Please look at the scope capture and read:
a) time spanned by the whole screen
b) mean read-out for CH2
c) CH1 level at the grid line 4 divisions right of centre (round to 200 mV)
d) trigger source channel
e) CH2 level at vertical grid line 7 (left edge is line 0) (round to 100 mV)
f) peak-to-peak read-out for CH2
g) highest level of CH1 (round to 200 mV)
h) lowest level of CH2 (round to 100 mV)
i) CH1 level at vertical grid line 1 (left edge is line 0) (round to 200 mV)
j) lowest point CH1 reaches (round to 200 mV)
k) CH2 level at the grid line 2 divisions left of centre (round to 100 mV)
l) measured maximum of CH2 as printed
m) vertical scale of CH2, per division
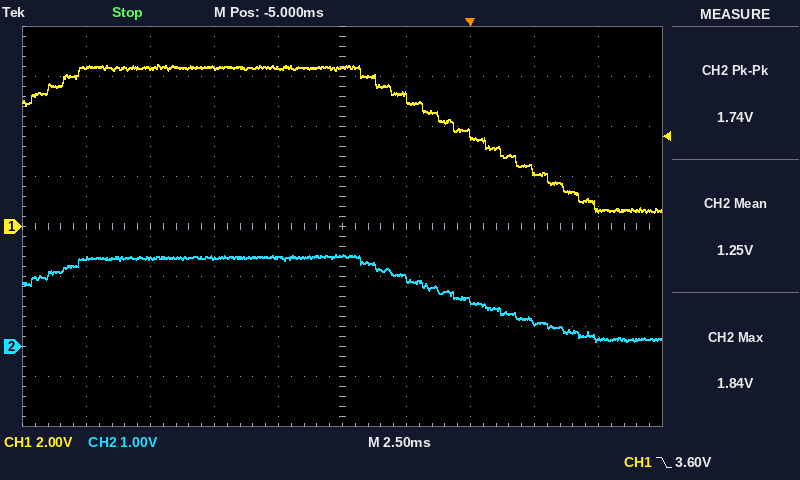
25 ms
1.25 V
600 mV
CH1
900 mV
1.74 V
6.4 V
100 mV
6.4 V
600 mV
1.8 V
1.84 V
1 V
